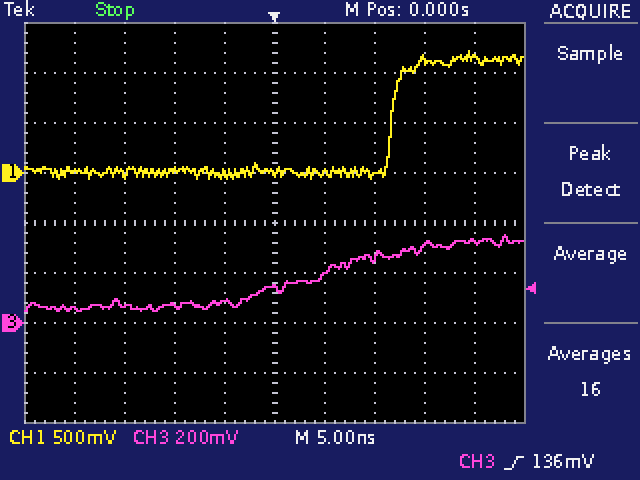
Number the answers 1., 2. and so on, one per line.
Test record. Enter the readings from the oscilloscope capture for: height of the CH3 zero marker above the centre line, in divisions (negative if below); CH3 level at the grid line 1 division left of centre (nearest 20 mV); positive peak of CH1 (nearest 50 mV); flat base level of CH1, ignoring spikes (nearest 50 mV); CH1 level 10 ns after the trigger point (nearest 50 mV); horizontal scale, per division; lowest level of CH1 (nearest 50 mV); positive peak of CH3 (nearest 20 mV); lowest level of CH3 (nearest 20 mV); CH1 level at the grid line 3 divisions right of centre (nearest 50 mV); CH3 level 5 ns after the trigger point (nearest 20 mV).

1. -2.0 div
2. 80 mV
3. 1.20 V
4. 0 mV
5. -50 mV
6. 5 ns
7. -50 mV
8. 360 mV
9. 40 mV
10. 1.15 V
11. 200 mV
